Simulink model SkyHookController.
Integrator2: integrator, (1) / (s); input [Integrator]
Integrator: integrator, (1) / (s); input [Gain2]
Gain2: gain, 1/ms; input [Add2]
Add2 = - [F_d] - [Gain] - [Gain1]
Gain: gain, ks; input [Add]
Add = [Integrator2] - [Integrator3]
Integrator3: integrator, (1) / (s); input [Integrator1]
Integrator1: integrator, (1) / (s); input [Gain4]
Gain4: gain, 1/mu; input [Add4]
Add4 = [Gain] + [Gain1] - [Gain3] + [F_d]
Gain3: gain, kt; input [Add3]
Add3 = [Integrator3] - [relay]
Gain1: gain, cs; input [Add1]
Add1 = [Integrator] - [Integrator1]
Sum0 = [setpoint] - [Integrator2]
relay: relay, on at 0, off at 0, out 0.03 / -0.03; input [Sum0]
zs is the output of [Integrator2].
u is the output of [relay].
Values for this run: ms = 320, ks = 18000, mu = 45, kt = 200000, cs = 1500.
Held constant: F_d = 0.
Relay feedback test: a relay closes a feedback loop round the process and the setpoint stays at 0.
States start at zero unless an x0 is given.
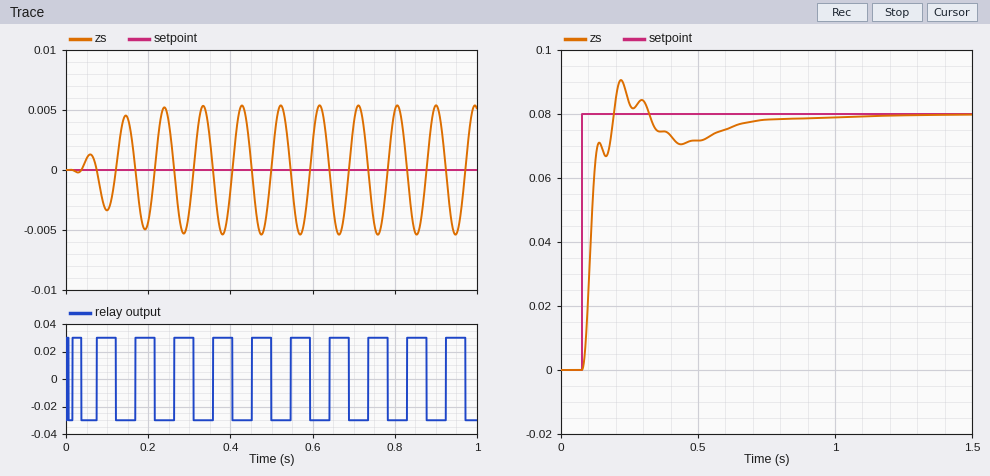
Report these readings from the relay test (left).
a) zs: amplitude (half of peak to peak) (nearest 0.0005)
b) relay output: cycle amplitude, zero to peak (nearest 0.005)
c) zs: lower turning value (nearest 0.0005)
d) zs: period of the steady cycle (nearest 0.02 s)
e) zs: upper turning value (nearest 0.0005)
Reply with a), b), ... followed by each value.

a) 0.0055
b) 0.030
c) -0.0055
d) 0.10 s
e) 0.0055
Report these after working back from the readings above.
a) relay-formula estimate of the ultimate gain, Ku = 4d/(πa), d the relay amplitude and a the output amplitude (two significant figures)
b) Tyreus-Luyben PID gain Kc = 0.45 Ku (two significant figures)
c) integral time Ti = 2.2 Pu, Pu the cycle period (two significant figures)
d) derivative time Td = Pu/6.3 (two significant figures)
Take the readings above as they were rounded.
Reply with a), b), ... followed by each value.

a) 6.9
b) 3.1
c) 0.22 s
d) 0.016 s
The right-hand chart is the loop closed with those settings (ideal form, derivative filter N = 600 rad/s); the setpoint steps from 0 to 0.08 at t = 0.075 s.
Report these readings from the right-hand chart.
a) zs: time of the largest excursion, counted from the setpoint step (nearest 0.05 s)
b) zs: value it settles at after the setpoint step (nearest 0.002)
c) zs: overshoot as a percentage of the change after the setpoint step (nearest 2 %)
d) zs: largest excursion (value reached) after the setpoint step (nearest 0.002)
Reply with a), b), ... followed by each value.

a) 0.15 s
b) 0.080
c) 14 %
d) 0.090
